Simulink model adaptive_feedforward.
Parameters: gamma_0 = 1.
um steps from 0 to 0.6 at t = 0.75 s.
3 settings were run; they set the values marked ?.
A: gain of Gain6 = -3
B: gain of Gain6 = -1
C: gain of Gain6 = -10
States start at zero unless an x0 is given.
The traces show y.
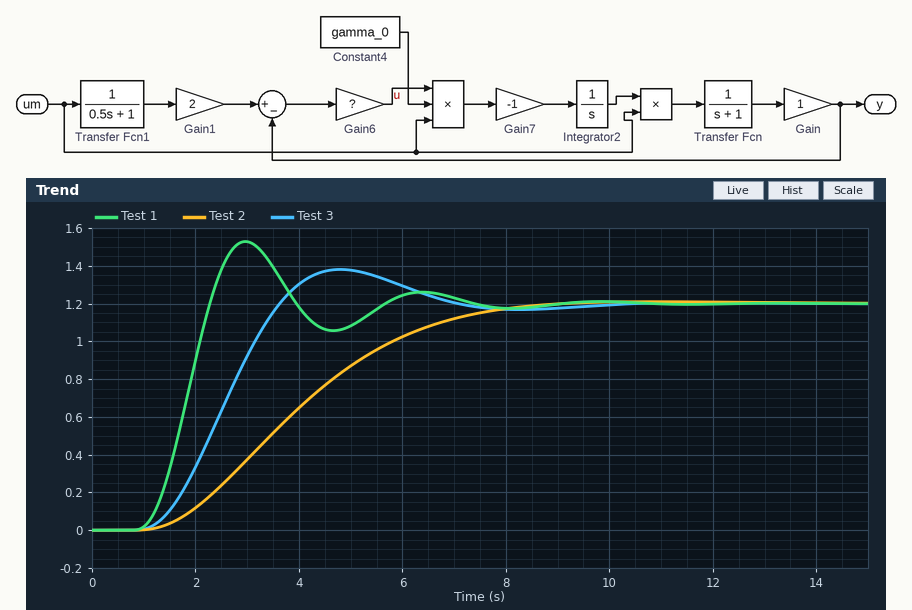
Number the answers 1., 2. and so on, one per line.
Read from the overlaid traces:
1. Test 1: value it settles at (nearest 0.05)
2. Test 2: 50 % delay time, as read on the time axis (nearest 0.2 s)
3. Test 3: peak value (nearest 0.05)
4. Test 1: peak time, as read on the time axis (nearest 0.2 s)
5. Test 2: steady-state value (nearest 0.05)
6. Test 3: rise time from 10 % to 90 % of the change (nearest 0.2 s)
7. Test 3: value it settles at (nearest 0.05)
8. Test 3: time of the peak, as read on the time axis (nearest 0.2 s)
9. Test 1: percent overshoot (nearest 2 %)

1. 1.20
2. 3.8 s
3. 1.40
4. 3.0 s
5. 1.20
6. 1.8 s
7. 1.20
8. 4.8 s
9. 28 %
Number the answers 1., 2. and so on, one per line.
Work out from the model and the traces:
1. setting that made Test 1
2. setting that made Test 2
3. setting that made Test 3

1. C
2. B
3. A
